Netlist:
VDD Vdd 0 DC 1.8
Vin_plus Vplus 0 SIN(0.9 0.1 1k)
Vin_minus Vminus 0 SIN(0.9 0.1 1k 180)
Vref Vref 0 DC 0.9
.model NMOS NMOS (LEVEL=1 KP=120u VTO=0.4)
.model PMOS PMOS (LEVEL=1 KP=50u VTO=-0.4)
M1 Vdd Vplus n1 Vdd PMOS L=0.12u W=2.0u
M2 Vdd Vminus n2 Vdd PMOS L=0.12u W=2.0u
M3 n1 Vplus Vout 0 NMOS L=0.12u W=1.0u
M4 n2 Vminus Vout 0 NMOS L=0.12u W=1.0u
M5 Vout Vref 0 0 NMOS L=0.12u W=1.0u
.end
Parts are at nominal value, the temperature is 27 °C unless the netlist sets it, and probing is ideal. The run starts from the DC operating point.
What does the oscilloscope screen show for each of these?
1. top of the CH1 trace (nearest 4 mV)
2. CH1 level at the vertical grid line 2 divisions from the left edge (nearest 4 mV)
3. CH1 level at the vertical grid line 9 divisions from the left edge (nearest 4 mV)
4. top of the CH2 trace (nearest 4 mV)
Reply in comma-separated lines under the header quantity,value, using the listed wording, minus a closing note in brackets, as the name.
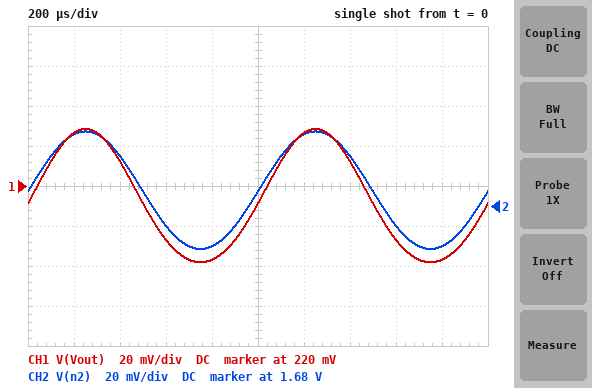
quantity,value
top of the CH1 trace,248 mV
CH1 level at the vertical grid line 2 divisions from the left edge,232 mV
CH1 level at the vertical grid line 9 divisions from the left edge,184 mV
top of the CH2 trace,1.716 V
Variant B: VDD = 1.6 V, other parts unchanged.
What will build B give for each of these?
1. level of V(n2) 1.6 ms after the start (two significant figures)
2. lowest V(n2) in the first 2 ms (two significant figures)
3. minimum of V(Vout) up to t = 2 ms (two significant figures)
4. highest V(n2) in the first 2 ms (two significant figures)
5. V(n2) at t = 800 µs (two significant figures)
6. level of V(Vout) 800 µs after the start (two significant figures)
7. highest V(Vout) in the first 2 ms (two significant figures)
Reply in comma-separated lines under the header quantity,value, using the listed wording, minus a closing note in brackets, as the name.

quantity,value
level of V(n2) 1.6 ms after the start,330 mV
lowest V(n2) in the first 2 ms,240 mV
minimum of V(Vout) up to t = 2 ms,120 mV
highest V(n2) in the first 2 ms,370 mV
V(n2) at t = 800 µs,300 mV
level of V(Vout) 800 µs after the start,160 mV
highest V(Vout) in the first 2 ms,200 mV
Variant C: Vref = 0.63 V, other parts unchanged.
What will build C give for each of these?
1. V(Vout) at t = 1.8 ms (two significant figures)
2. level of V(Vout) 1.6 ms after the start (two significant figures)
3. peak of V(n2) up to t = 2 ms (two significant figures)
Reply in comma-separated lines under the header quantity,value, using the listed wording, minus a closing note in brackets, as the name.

quantity,value
V(Vout) at t = 1.8 ms,300 mV
level of V(Vout) 1.6 ms after the start,310 mV
peak of V(n2) up to t = 2 ms,1.8 V
